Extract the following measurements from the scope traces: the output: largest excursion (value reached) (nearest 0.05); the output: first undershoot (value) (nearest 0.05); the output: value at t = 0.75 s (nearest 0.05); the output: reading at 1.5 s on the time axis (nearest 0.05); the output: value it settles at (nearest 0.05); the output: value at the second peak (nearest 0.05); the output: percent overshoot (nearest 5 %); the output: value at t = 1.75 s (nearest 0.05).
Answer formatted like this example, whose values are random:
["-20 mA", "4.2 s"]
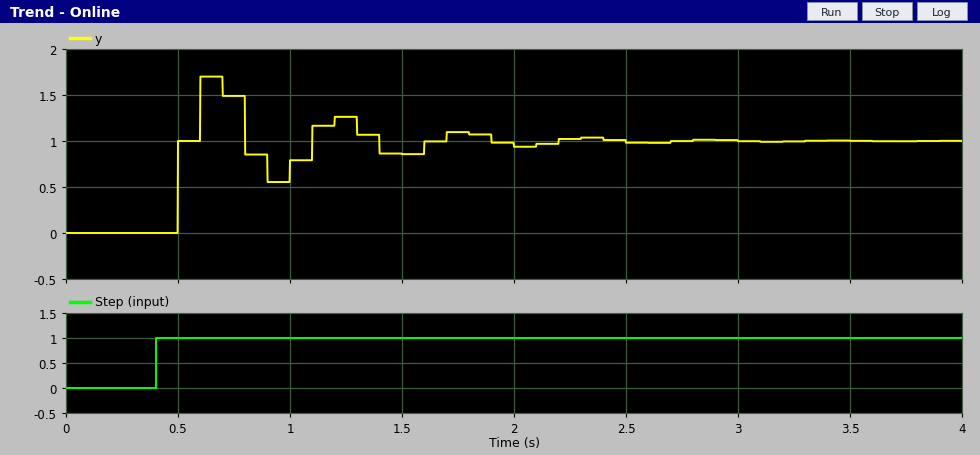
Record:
["1.70", "0.55", "1.50", "0.85", "1.00", "1.25", "70 %", "1.10"]
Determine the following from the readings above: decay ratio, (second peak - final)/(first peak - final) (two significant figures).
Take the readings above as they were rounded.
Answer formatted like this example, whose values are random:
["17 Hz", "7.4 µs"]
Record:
["0.36"]
